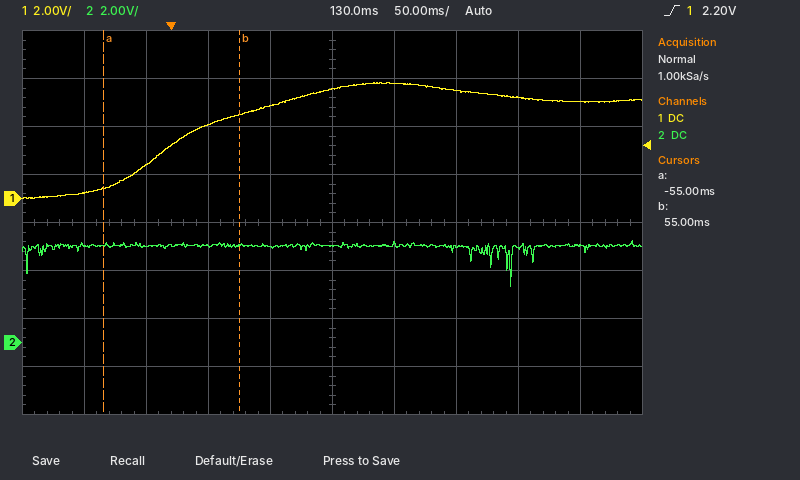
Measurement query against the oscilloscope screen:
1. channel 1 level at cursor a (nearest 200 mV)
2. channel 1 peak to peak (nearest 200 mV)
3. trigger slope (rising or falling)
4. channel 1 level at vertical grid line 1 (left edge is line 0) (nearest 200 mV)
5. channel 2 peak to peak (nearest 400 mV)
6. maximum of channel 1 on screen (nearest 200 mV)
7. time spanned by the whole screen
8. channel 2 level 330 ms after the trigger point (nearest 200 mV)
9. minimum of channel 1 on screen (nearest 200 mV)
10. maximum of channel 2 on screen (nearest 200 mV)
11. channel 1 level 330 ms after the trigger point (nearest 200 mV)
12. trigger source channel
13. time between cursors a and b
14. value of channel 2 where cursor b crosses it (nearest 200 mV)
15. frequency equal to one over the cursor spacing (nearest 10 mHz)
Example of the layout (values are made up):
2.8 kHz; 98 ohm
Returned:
400 mV; 4.8 V; rising; 200 mV; 2.0 V; 4.8 V; 500 ms; 4.0 V; 0.0 V; 4.2 V; 4.0 V; channel 1; 110 ms; 4.0 V; 9.09 Hz
